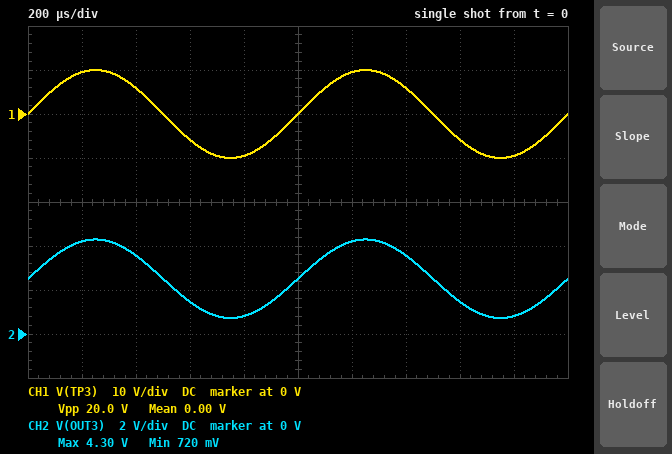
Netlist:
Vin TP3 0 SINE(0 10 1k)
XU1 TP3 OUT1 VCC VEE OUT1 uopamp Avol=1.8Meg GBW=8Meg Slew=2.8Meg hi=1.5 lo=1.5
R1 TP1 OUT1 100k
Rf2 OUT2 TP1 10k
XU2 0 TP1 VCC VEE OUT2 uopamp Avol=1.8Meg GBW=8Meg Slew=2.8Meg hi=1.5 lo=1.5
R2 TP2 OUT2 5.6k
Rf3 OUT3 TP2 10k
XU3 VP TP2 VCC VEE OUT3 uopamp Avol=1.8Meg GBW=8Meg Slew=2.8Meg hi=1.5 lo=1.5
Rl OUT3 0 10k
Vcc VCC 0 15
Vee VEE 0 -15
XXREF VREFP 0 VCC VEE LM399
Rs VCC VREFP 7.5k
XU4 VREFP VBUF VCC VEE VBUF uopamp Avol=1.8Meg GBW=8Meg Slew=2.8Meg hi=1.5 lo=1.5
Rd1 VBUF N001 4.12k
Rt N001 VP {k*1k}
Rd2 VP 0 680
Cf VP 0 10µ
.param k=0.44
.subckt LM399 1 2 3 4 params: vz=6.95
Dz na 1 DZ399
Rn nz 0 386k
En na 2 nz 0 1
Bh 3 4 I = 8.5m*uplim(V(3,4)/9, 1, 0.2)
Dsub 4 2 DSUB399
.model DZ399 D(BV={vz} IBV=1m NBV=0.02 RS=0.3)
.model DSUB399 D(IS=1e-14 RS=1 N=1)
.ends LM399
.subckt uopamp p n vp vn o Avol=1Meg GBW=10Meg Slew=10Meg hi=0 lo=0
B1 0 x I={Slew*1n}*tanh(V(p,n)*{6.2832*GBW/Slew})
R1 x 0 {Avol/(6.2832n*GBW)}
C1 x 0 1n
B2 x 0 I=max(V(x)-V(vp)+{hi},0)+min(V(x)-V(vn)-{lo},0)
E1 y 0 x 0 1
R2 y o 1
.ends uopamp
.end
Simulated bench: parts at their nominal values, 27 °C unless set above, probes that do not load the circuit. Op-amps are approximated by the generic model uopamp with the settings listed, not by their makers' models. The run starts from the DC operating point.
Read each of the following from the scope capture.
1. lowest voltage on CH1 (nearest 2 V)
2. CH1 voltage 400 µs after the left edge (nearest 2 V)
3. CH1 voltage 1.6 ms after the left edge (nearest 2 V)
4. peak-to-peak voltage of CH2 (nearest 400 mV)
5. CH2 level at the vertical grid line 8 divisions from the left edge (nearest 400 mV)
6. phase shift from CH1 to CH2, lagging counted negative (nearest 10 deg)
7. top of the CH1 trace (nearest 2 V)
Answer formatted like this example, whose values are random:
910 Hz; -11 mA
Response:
-10 V; 6 V; -6 V; 3.6 V; 1.6 V; 0 deg; 10 V
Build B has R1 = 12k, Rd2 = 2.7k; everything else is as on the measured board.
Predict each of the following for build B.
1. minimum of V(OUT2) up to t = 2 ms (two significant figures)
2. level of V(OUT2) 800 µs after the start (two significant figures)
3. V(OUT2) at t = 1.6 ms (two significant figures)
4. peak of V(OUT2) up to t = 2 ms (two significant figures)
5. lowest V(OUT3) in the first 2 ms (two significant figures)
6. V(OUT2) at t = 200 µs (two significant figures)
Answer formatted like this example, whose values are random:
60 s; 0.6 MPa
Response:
-8.3 V; 7.9 V; 4.9 V; 8.3 V; -7.7 V; -7.9 V
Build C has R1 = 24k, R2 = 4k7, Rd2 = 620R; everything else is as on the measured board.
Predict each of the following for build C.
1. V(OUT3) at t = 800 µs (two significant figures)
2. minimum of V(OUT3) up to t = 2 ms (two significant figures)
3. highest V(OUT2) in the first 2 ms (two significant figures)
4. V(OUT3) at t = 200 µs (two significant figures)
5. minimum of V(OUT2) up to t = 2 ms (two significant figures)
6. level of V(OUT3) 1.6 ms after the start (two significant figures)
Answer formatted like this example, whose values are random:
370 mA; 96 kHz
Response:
-5.8 V; -6.3 V; 4.2 V; 11 V; -4.2 V; -2.6 V
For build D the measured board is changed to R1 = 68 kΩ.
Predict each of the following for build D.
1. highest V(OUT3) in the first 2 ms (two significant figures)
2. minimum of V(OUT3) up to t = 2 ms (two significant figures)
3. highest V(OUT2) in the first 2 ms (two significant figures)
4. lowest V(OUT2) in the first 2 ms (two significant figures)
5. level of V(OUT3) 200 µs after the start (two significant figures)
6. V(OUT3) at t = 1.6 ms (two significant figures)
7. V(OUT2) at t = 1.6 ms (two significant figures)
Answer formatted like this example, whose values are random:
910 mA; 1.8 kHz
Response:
5.1 V; -110 mV; 1.5 V; -1.5 V; 5.0 V; 970 mV; 860 mV
